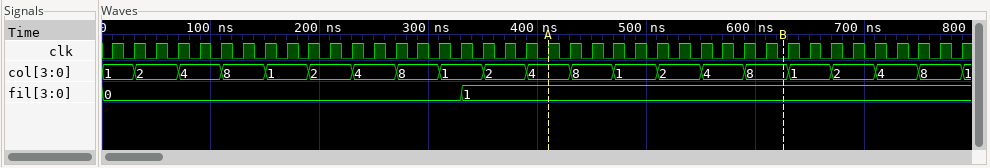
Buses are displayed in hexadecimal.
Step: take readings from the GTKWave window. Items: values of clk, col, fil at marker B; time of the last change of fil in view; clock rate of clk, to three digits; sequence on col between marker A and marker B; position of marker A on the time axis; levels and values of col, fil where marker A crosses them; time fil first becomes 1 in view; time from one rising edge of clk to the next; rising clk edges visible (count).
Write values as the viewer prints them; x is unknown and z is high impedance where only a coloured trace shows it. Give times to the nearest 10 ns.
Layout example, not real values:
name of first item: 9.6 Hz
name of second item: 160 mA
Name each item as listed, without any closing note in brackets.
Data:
values of clk, col, fil at marker B: clk=0, col=8, fil=1
time of the last change of fil in view: 330 ns
clock rate of clk, to three digits: 50.0 MHz
sequence on col between marker A and marker B: 4, 8, 1, 2, 4, 8
position of marker A on the time axis: 410 ns
levels and values of col, fil where marker A crosses them: col=4, fil=1
time fil first becomes 1 in view: 330 ns
time from one rising edge of clk to the next: 20 ns
rising clk edges visible: 40
